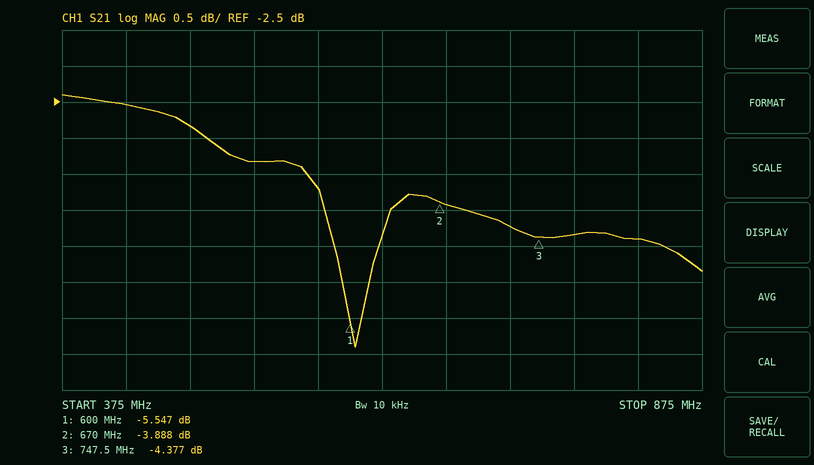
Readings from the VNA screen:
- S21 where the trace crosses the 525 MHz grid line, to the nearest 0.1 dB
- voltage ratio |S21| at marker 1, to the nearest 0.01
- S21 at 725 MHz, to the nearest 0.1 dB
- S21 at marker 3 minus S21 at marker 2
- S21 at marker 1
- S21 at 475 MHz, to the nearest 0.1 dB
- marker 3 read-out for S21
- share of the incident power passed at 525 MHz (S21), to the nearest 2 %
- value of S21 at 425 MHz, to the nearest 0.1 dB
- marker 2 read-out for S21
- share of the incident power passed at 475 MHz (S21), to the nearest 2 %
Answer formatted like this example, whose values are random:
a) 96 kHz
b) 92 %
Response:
a) -3.3 dB
b) 0.53
c) -4.2 dB
d) -0.489 dB
e) -5.547 dB
f) -2.8 dB
g) -4.377 dB
h) 46 %
i) -2.5 dB
j) -3.888 dB
k) 52 %
